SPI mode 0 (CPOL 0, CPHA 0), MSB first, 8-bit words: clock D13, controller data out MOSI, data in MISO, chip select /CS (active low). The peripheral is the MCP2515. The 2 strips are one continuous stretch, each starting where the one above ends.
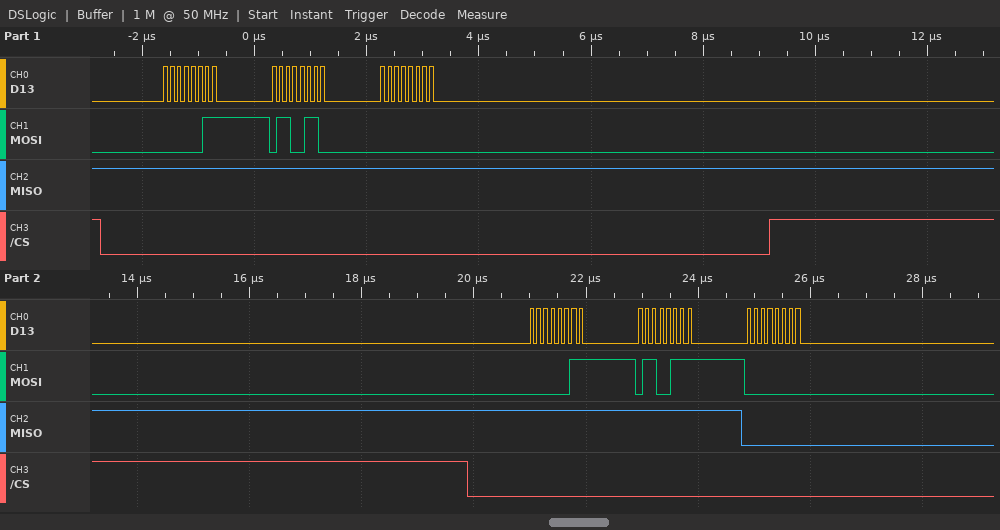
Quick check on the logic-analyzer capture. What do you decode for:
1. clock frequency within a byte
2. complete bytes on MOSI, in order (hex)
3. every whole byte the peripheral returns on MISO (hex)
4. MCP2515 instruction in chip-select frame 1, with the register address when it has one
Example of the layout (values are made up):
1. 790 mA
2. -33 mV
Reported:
1. 8 MHz
2. 03 66 00 03 67 00
3. FF FF FF FF FF 00
4. READ 0x66
